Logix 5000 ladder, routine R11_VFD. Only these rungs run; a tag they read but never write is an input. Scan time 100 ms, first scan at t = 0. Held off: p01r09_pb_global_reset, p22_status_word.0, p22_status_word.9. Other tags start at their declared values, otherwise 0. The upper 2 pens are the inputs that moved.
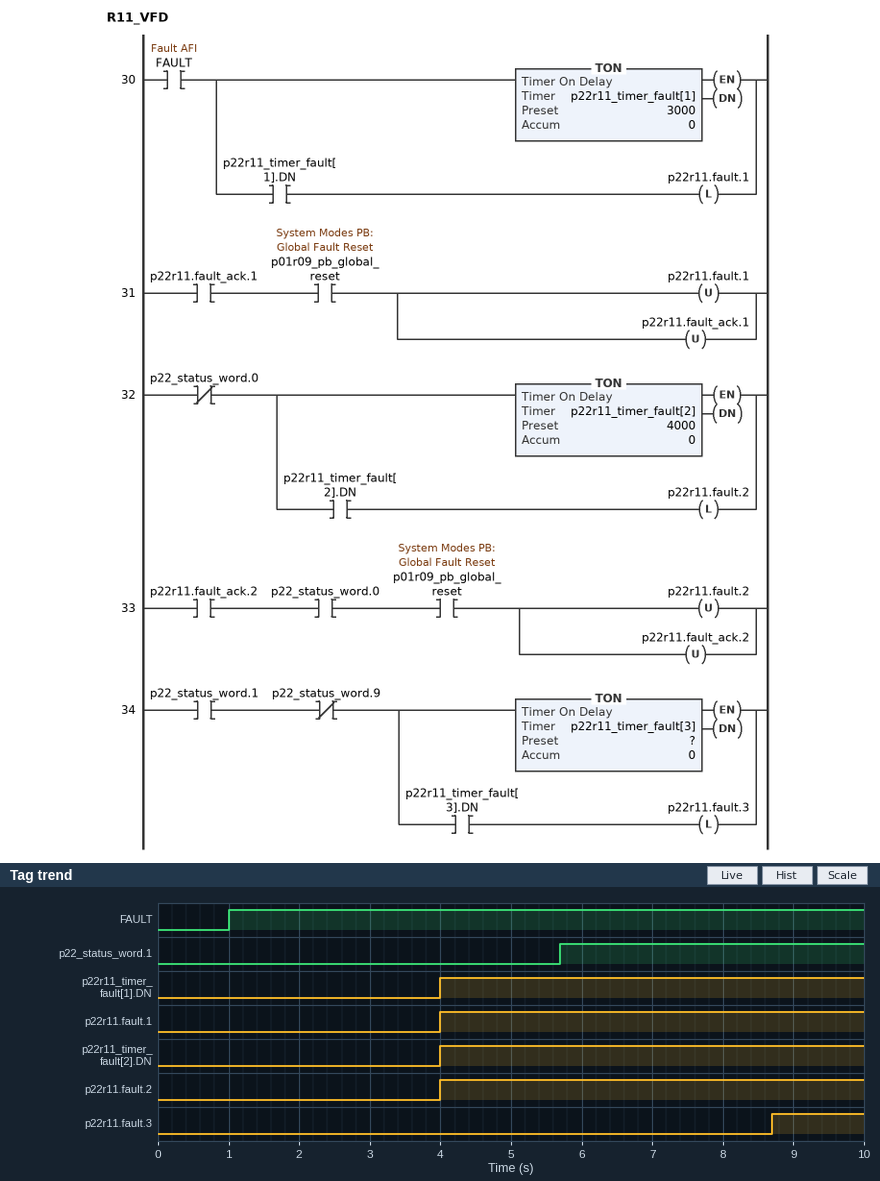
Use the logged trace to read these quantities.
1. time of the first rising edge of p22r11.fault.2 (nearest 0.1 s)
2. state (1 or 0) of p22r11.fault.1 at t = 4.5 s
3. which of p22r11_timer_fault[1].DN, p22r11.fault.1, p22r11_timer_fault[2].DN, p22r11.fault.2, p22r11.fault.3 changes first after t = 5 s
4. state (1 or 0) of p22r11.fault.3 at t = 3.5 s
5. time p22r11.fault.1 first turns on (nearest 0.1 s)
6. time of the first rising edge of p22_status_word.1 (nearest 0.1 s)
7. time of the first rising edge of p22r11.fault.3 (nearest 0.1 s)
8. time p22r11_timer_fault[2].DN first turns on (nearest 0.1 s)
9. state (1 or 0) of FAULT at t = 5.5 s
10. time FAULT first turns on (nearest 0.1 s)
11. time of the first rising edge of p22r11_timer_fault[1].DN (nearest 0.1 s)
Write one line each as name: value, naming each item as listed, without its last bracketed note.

time of the first rising edge of p22r11.fault.2: 4.0 s
state (1 or 0) of p22r11.fault.1 at t = 4.5 s: 1
which of p22r11_timer_fault[1].DN, p22r11.fault.1, p22r11_timer_fault[2].DN, p22r11.fault.2, p22r11.fault.3 changes first after t = 5 s: p22r11.fault.3
state (1 or 0) of p22r11.fault.3 at t = 3.5 s: 0
time p22r11.fault.1 first turns on: 4.0 s
time of the first rising edge of p22_status_word.1: 5.7 s
time of the first rising edge of p22r11.fault.3: 8.7 s
time p22r11_timer_fault[2].DN first turns on: 4.0 s
state (1 or 0) of FAULT at t = 5.5 s: 1
time FAULT first turns on: 1.0 s
time of the first rising edge of p22r11_timer_fault[1].DN: 4.0 s
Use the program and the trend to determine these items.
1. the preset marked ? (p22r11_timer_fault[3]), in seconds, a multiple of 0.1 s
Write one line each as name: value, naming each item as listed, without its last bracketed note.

the preset marked ? (p22r11_timer_fault[3]), in seconds, a multiple of 0.1 s: 3.0 s
